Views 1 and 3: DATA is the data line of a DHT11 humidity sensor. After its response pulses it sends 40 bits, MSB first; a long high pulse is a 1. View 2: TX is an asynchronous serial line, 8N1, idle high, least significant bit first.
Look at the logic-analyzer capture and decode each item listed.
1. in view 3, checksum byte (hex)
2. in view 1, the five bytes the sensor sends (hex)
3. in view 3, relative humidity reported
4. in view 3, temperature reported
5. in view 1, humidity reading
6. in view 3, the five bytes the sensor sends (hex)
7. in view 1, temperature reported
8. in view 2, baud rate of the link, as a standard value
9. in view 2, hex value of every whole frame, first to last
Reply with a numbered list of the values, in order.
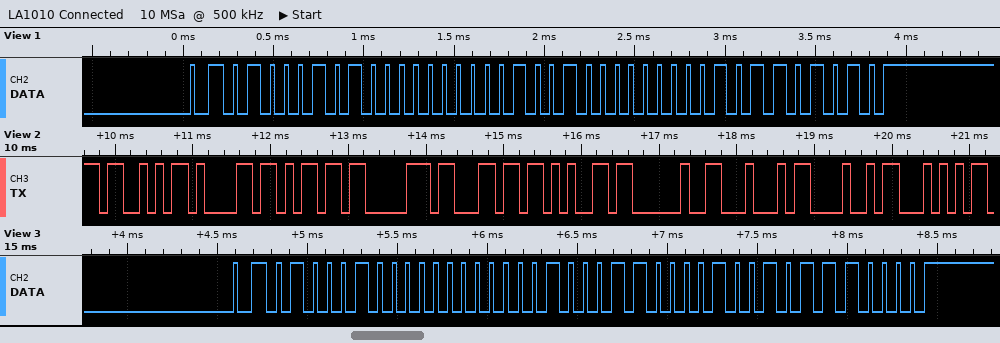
1. 0x70
2. 45 00 24 01 6A
3. 68 %
4. 35.9 °C
5. 69 %
6. 44 00 23 09 70
7. 36.1 °C
8. 9600 baud
9. 53 61 6D 70 6C 65 20 44 48 54
